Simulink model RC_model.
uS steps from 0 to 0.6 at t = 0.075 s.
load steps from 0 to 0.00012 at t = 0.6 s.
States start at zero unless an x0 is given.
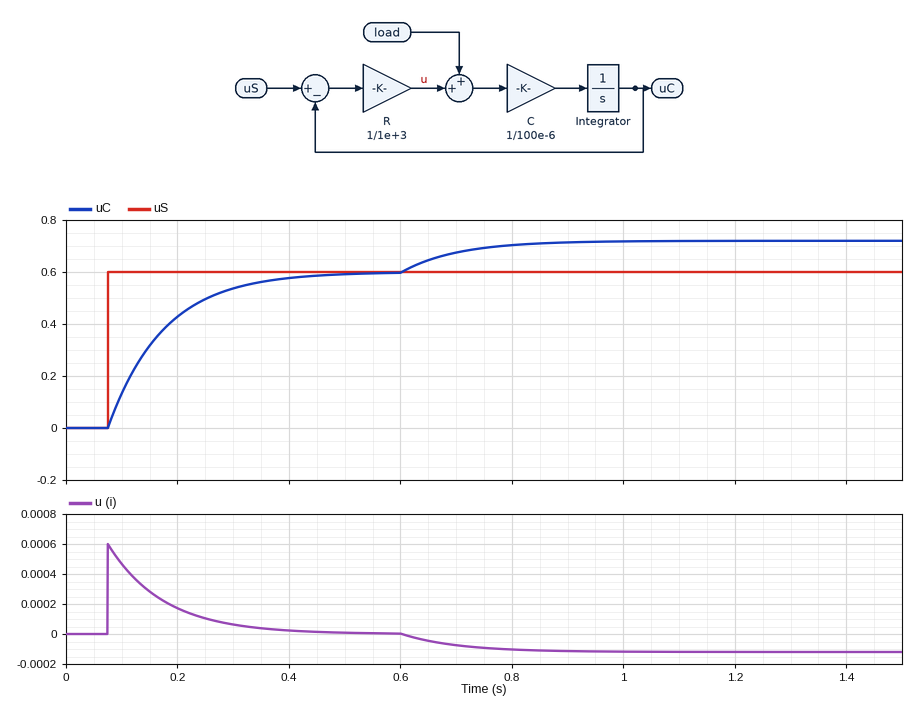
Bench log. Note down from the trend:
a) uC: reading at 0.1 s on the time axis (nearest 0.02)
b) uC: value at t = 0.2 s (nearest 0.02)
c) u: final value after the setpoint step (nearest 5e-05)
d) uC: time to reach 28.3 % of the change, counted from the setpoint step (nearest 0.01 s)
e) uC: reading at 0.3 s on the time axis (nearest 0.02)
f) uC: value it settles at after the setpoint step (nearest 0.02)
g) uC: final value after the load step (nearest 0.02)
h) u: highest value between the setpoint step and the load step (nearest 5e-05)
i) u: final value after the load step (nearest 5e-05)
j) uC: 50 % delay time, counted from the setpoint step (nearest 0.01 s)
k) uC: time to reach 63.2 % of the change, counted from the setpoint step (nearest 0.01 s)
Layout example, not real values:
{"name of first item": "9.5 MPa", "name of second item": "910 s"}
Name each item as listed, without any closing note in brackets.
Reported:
{"uC: reading at 0.1 s on the time axis": "0.14", "uC: value at t = 0.2 s": "0.42", "u: final value after the setpoint step": "0.00000", "uC: time to reach 28.3 % of the change, counted from the setpoint step": "0.03 s", "uC: reading at 0.3 s on the time axis": "0.54", "uC: value it settles at after the setpoint step": "0.60", "uC: final value after the load step": "0.72", "u: highest value between the setpoint step and the load step": "0.00060", "u: final value after the load step": "-0.00010", "uC: 50 % delay time, counted from the setpoint step": "0.07 s", "uC: time to reach 63.2 % of the change, counted from the setpoint step": "0.10 s"}
